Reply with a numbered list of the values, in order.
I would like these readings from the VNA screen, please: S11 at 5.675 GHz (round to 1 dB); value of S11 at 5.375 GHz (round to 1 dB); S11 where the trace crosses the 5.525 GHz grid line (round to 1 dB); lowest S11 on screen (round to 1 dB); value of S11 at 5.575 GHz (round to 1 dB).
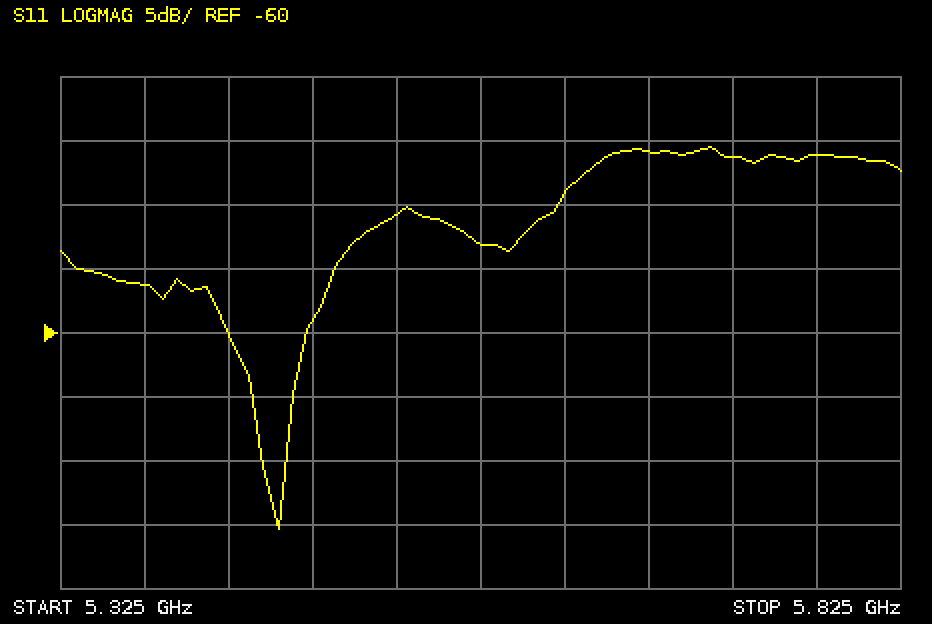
1. -46 dB
2. -56 dB
3. -51 dB
4. -75 dB
5. -53 dB
